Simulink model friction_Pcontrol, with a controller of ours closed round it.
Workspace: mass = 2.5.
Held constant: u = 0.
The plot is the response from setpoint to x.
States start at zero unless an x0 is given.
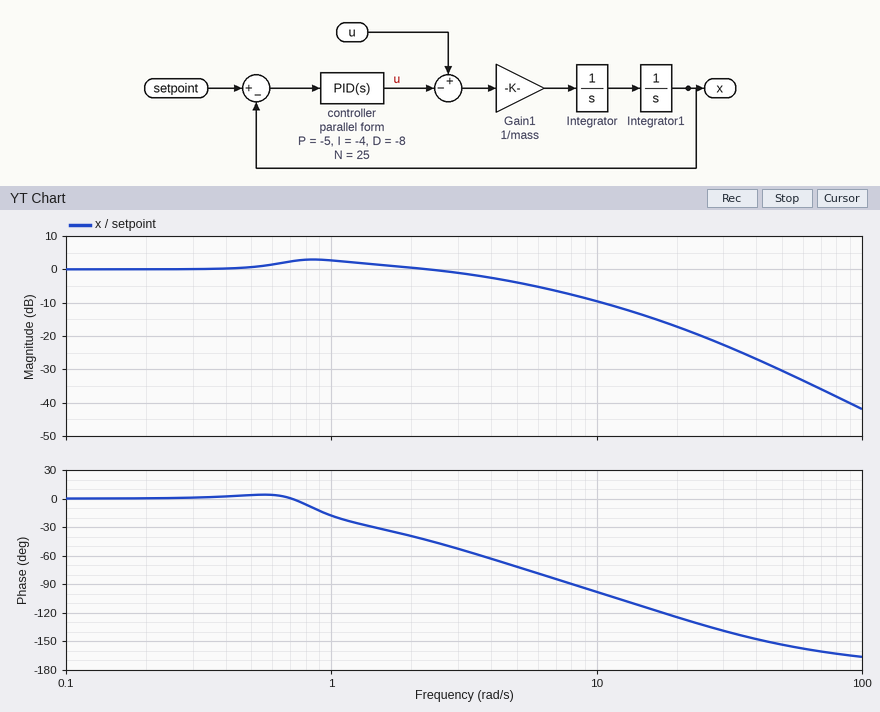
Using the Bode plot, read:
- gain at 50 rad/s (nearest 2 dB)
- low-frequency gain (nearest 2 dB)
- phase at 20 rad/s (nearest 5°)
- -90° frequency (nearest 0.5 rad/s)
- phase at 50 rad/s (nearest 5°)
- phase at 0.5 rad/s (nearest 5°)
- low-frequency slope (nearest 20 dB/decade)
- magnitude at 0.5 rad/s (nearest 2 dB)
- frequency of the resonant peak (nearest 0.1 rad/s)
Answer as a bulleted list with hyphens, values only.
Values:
- -30 dB
- 0 dB
- -125°
- 8.0 rad/s
- -155°
- 5°
- 0 dB/decade
- 0 dB
- 0.9 rad/s
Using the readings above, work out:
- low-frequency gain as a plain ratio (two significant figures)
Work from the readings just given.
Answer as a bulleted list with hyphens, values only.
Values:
- 1.0
